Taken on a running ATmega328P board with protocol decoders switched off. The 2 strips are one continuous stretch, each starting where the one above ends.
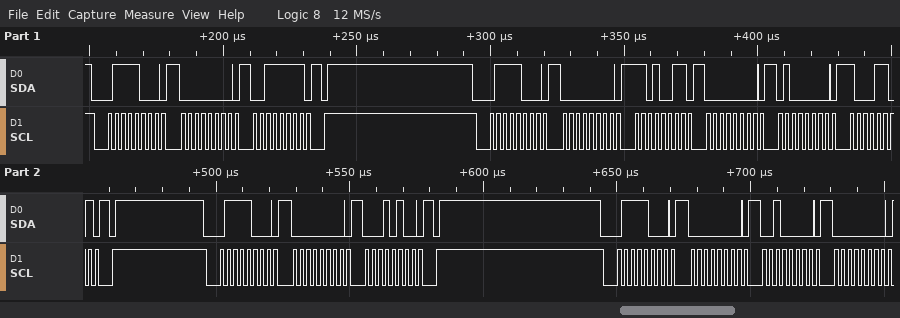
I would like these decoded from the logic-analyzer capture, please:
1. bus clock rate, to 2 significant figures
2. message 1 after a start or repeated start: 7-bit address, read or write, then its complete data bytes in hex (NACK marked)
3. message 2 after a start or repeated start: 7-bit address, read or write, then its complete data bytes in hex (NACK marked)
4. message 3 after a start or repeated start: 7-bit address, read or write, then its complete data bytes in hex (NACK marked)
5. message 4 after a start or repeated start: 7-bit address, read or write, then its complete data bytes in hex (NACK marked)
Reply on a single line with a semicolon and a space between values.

400 kHz; 0x3C write: 00 3F; 0x3C write: 00 D3 00 40 8D; 0x3C write: 00 14; 0x3C write: 00 20 00
